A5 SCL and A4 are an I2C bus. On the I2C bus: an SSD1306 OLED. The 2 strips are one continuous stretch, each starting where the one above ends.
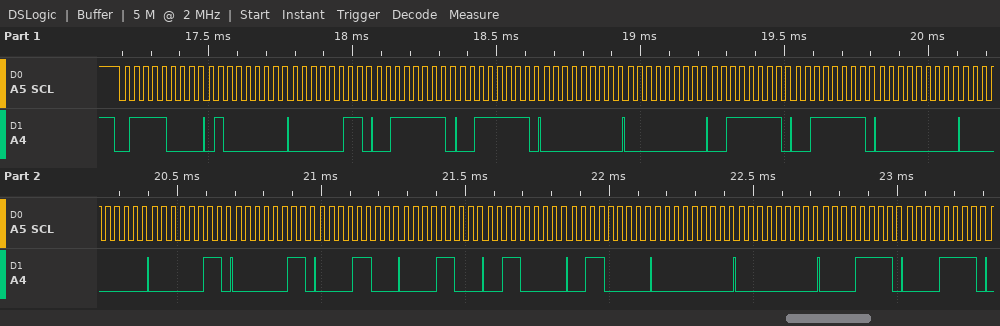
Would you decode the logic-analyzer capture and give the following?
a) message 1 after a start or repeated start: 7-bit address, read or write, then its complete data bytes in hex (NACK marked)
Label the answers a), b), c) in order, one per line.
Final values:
a) 0x3C write: 40 03 3F 3F 00 00 3F 3F 00 00 03 03 0C 0C 30 30 00 00 0F 0F
